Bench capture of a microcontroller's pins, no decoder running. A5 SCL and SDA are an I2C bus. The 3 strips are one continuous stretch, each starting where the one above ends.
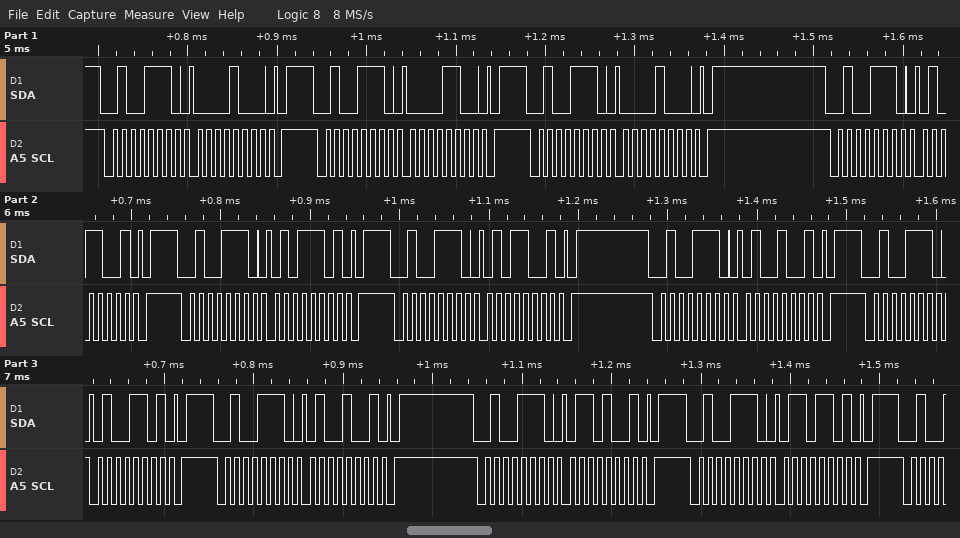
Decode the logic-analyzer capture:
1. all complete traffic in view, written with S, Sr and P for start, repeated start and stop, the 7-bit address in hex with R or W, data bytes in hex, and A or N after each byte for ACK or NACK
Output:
S 27W A 08 A P S 27W A 0C A P S 27W A 08 A P S 27W A 59 A P S 27W A 5D A P S 27W A 59 A P S 27W A 49 A P S 27W A 4D A P S 27W A 49 A P S 27W A 69 A P S 27W A 6D A P
